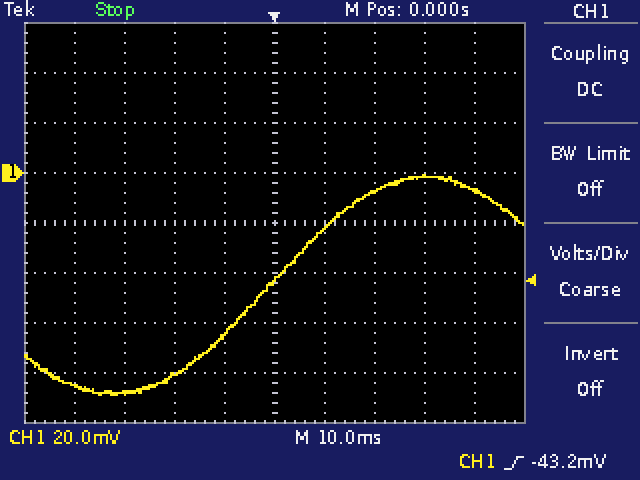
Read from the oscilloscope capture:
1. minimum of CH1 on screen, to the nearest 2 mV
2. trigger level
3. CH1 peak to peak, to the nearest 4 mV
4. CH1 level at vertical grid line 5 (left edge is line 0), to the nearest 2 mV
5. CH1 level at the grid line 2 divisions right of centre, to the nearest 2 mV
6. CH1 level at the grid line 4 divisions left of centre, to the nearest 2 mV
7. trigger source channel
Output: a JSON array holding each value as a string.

["-88 mV", "-43.2 mV", "88 mV", "-44 mV", "-8 mV", "-84 mV", "CH1"]
